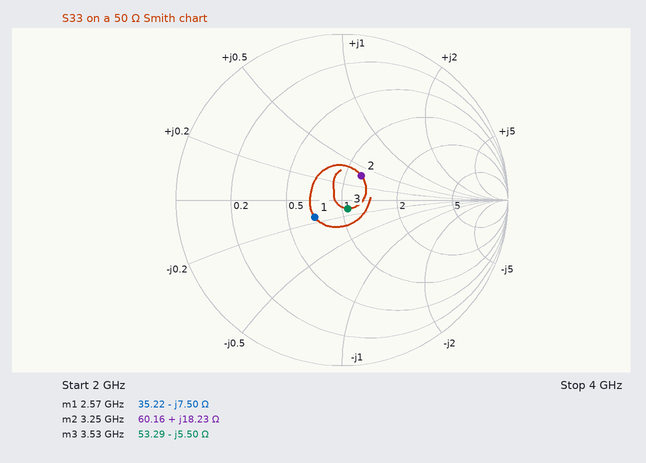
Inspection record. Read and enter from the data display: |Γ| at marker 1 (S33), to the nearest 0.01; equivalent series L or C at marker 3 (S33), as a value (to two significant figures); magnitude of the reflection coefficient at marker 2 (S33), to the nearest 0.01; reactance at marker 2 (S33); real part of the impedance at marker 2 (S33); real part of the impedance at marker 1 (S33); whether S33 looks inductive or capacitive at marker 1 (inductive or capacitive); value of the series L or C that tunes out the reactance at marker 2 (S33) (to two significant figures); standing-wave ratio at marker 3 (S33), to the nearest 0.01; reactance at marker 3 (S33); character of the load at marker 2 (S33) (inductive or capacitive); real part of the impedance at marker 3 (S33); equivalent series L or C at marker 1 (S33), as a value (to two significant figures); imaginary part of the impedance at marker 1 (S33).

0.19
8.2 pF
0.19
+18.23 Ω
60.16 Ω
35.22 Ω
capacitive
2.7 pF
1.13
-5.50 Ω
inductive
53.29 Ω
8.3 pF
-7.50 Ω
